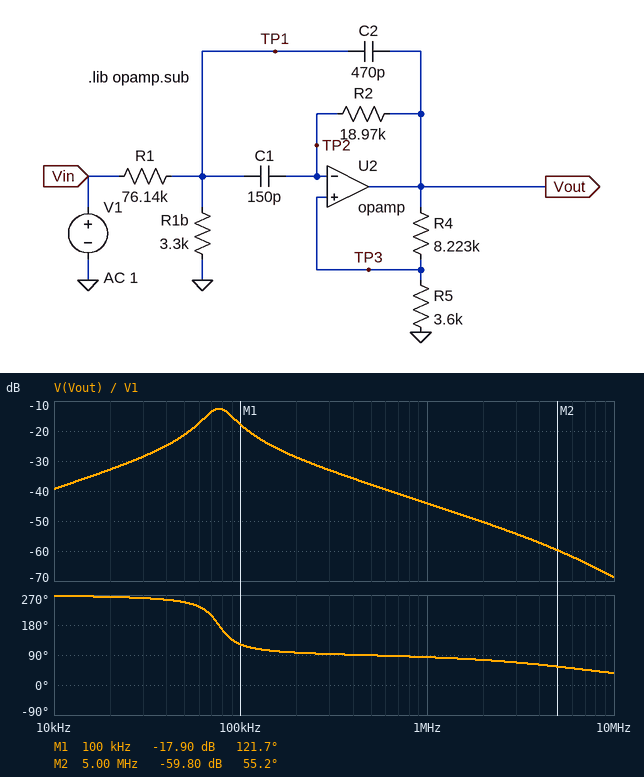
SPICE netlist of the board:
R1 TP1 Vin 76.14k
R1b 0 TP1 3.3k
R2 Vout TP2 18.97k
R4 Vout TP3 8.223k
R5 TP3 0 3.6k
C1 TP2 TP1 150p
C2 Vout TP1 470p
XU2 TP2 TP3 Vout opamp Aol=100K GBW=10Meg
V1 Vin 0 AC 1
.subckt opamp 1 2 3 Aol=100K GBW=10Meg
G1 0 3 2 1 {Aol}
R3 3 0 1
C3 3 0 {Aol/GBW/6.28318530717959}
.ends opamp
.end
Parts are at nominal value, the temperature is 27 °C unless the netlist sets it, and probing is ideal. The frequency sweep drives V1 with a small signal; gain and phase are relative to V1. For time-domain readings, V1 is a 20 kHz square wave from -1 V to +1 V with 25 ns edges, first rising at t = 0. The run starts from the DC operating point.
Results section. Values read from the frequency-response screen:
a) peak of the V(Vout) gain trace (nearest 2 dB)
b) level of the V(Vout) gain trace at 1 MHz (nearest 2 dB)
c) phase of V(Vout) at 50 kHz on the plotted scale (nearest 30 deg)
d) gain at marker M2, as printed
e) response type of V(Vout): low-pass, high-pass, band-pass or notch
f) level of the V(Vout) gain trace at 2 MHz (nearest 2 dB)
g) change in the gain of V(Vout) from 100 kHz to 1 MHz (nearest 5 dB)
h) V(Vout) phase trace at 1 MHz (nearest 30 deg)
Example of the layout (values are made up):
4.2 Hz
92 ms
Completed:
-12 dB
-44 dB
240 deg
-59.80 dB
band-pass
-50 dB
-25 dB
90 deg
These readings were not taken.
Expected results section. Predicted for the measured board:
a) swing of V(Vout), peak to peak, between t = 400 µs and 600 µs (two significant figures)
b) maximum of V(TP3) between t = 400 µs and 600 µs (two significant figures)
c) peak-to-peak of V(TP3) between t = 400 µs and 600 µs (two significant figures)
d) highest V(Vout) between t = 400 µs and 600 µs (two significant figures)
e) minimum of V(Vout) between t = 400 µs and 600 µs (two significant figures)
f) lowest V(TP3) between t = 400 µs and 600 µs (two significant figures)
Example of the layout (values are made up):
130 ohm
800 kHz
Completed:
240 mV
36 mV
72 mV
120 mV
-120 mV
-36 mV
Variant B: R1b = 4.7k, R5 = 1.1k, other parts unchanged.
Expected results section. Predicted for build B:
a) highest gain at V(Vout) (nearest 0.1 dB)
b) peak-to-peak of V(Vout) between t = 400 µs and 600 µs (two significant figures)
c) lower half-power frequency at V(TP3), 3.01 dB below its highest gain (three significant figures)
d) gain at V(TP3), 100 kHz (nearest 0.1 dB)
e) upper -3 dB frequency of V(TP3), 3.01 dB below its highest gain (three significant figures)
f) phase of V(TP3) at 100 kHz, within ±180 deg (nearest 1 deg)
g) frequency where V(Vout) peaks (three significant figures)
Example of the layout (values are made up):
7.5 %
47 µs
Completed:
-22.0 dB
170 mV
40.8 kHz
-43.2 dB
104 kHz
137 deg
65.1 kHz
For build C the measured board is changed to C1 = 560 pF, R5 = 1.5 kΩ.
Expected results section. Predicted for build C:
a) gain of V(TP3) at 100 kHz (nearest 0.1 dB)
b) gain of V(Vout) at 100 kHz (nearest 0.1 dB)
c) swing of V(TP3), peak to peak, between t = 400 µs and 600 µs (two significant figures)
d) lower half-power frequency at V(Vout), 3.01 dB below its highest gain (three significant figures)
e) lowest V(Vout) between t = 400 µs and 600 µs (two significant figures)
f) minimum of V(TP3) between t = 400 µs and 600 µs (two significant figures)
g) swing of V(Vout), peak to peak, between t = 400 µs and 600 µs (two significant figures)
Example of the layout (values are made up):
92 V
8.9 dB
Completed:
-40.6 dB
-24.3 dB
47 mV
33.7 kHz
-150 mV
-24 mV
310 mV
